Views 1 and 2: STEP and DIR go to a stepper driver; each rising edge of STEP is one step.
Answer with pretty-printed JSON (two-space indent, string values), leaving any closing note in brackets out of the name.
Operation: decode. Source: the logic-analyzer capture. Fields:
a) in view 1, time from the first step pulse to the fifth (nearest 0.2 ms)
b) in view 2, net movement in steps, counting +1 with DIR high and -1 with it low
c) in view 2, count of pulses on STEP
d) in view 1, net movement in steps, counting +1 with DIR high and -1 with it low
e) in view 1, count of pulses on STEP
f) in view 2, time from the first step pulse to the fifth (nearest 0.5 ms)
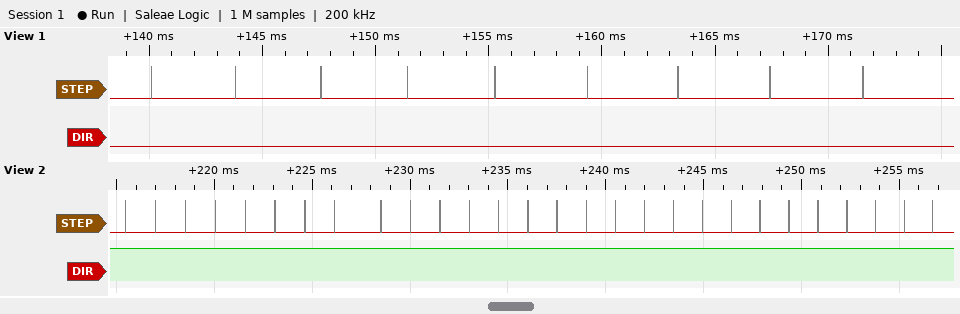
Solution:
{
  "in view 1, time from the first step pulse to the fifth": "15.2 ms",
  "in view 2, net movement in steps, counting +1 with DIR high and -1 with it low": "+28",
  "in view 2, count of pulses on STEP": "28",
  "in view 1, net movement in steps, counting +1 with DIR high and -1 with it low": "-9",
  "in view 1, count of pulses on STEP": "9",
  "in view 2, time from the first step pulse to the fifth": "6.0 ms"
}
